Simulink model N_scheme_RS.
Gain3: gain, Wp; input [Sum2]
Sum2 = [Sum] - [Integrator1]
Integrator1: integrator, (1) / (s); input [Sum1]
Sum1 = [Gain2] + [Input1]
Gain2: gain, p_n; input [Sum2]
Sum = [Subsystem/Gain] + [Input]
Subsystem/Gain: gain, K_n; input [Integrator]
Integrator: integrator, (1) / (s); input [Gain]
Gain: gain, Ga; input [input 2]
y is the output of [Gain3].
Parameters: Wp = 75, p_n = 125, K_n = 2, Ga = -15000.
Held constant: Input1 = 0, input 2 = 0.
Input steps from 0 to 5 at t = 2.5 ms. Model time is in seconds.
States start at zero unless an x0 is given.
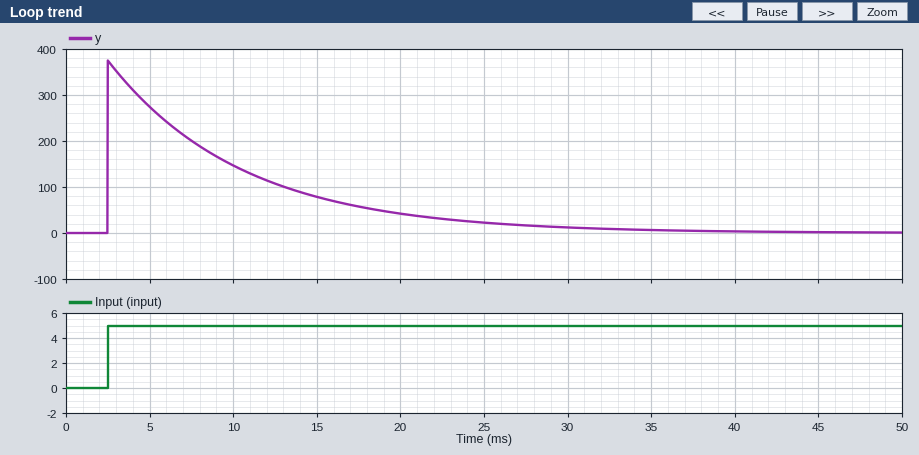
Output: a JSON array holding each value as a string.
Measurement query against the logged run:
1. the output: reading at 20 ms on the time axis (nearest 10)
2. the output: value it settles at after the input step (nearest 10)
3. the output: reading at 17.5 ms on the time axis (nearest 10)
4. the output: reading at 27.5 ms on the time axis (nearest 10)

["40", "0", "60", "20"]
